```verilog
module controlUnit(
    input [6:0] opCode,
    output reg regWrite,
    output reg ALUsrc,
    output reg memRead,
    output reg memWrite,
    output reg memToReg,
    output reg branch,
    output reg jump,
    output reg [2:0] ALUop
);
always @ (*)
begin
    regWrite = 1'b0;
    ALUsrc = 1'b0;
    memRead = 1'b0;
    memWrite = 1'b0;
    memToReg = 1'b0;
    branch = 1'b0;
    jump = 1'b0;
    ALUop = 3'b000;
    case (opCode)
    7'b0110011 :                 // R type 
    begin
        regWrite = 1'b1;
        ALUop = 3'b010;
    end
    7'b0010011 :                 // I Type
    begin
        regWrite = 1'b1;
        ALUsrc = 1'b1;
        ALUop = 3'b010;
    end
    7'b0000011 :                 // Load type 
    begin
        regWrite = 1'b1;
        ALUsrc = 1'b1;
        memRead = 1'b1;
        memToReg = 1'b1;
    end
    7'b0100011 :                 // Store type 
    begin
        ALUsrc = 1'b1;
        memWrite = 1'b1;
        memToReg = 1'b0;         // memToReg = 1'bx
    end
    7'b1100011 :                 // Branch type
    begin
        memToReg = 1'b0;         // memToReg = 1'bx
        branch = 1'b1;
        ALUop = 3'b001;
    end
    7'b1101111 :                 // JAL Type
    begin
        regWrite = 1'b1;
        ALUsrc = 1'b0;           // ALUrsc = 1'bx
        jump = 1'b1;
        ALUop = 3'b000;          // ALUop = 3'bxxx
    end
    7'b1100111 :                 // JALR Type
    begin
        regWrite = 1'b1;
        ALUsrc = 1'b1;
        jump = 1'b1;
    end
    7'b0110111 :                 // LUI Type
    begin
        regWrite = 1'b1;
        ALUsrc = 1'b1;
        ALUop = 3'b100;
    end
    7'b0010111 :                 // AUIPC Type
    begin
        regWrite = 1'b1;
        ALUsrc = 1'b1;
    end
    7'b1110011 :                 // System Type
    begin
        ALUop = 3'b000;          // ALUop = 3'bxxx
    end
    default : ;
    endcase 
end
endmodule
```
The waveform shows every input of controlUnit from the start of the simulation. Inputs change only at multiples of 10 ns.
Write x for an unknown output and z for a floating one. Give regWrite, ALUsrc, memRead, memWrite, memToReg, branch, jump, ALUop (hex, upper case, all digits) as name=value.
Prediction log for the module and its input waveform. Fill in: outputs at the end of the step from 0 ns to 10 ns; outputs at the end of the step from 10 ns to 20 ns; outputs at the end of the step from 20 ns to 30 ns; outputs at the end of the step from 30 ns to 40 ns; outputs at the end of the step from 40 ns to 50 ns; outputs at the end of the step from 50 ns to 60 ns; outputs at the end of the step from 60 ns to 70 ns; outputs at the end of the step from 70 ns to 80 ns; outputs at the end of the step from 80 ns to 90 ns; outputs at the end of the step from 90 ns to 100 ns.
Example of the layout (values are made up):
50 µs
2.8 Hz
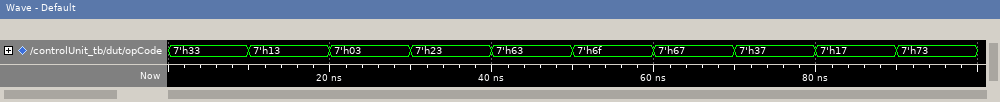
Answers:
regWrite=1, ALUsrc=0, memRead=0, memWrite=0, memToReg=0, branch=0, jump=0, ALUop=2
regWrite=1, ALUsrc=1, memRead=0, memWrite=0, memToReg=0, branch=0, jump=0, ALUop=2
regWrite=1, ALUsrc=1, memRead=1, memWrite=0, memToReg=1, branch=0, jump=0, ALUop=0
regWrite=0, ALUsrc=1, memRead=0, memWrite=1, memToReg=0, branch=0, jump=0, ALUop=0
regWrite=0, ALUsrc=0, memRead=0, memWrite=0, memToReg=0, branch=1, jump=0, ALUop=1
regWrite=1, ALUsrc=0, memRead=0, memWrite=0, memToReg=0, branch=0, jump=1, ALUop=0
regWrite=1, ALUsrc=1, memRead=0, memWrite=0, memToReg=0, branch=0, jump=1, ALUop=0
regWrite=1, ALUsrc=1, memRead=0, memWrite=0, memToReg=0, branch=0, jump=0, ALUop=4
regWrite=1, ALUsrc=1, memRead=0, memWrite=0, memToReg=0, branch=0, jump=0, ALUop=0
regWrite=0, ALUsrc=0, memRead=0, memWrite=0, memToReg=0, branch=0, jump=0, ALUop=0
